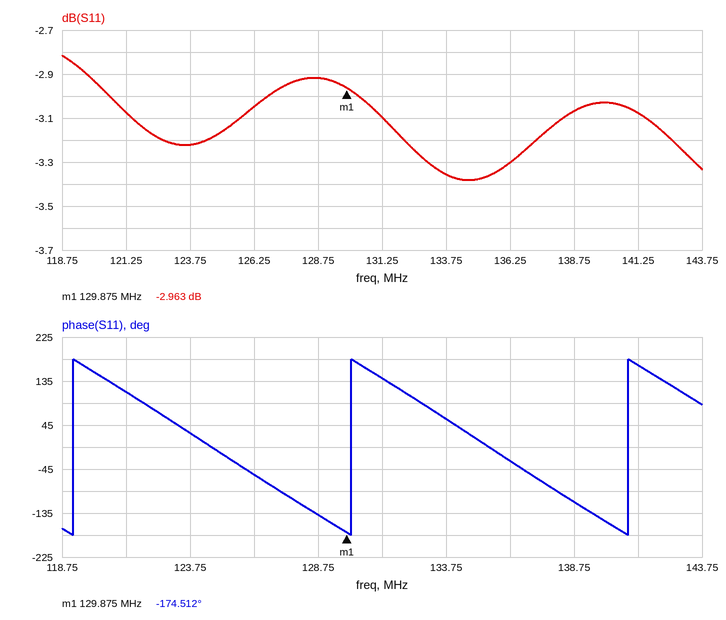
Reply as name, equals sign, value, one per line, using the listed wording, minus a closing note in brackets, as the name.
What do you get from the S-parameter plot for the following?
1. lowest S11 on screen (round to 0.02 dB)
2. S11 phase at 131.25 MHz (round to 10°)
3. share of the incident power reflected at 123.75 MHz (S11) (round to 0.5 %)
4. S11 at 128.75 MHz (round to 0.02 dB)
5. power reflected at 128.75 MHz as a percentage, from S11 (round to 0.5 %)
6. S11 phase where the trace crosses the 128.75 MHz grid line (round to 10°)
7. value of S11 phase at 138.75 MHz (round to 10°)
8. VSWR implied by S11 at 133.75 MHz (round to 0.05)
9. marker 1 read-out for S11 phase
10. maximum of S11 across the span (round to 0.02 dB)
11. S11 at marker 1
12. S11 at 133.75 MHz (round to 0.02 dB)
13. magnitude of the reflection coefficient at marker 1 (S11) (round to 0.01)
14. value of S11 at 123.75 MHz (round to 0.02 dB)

lowest S11 on screen = -3.38 dB
S11 phase at 131.25 MHz = 140°
share of the incident power reflected at 123.75 MHz (S11) = 47.5 %
S11 at 128.75 MHz = -2.92 dB
power reflected at 128.75 MHz as a percentage, from S11 = 51.0 %
S11 phase where the trace crosses the 128.75 MHz grid line = -140°
value of S11 phase at 138.75 MHz = -110°
VSWR implied by S11 at 133.75 MHz = 5.25
marker 1 read-out for S11 phase = -174.512°
maximum of S11 across the span = -2.82 dB
S11 at marker 1 = -2.963 dB
S11 at 133.75 MHz = -3.36 dB
magnitude of the reflection coefficient at marker 1 (S11) = 0.71
value of S11 at 123.75 MHz = -3.22 dB
